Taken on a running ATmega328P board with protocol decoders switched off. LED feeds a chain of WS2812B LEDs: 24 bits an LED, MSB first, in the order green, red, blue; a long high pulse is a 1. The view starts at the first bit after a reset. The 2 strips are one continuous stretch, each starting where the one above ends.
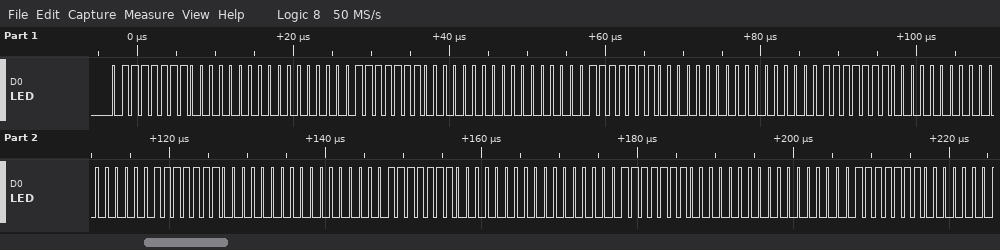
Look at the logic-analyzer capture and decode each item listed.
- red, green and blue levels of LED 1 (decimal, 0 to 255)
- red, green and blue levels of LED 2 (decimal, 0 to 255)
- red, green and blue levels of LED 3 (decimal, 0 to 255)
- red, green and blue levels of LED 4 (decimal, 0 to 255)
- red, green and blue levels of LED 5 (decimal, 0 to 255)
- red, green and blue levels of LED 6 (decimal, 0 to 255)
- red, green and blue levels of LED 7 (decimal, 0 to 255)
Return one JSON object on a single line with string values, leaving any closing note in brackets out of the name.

{"red, green and blue levels of LED 1": "0, 127, 0", "red, green and blue levels of LED 2": "0, 127, 0", "red, green and blue levels of LED 3": "0, 127, 0", "red, green and blue levels of LED 4": "0, 127, 0", "red, green and blue levels of LED 5": "0, 127, 0", "red, green and blue levels of LED 6": "0, 127, 0", "red, green and blue levels of LED 7": "0, 127, 0"}
